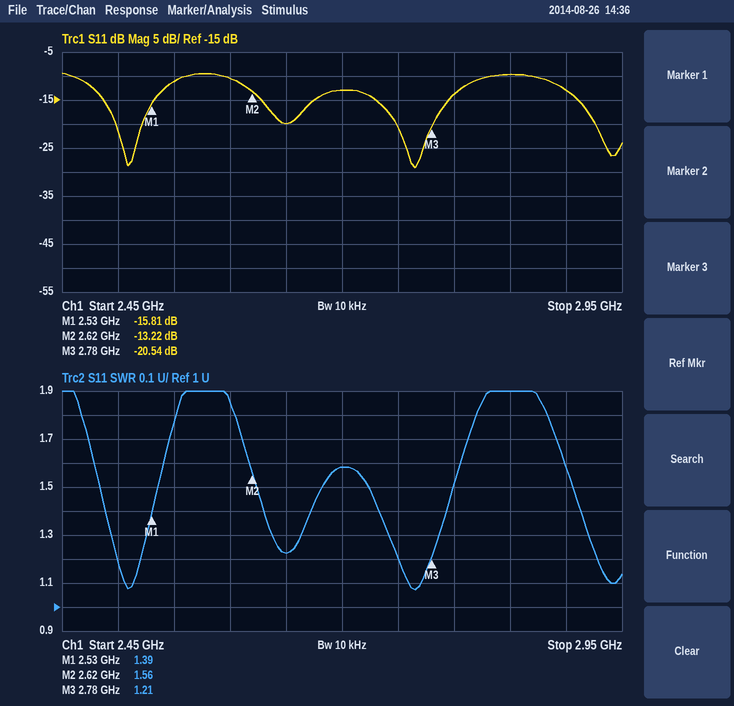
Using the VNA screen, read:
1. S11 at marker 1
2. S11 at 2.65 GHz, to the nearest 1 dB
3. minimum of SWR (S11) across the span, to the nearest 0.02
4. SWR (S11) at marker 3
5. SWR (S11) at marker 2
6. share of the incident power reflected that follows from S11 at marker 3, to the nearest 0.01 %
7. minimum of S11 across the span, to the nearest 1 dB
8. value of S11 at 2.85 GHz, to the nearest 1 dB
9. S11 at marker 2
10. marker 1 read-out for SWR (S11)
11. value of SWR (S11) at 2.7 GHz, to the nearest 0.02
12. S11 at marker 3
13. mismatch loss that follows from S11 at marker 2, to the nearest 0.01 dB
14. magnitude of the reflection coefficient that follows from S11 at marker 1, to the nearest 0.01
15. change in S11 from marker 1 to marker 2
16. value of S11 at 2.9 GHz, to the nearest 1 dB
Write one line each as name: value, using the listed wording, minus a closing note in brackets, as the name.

S11 at marker 1: -15.81 dB
S11 at 2.65 GHz, to the nearest 1 dB: -20 dB
minimum of SWR (S11) across the span, to the nearest 0.02: 1.08
SWR (S11) at marker 3: 1.21
SWR (S11) at marker 2: 1.56
share of the incident power reflected that follows from S11 at marker 3, to the nearest 0.01 %: 0.88 %
minimum of S11 across the span, to the nearest 1 dB: -29 dB
value of S11 at 2.85 GHz, to the nearest 1 dB: -10 dB
S11 at marker 2: -13.22 dB
marker 1 read-out for SWR: 1.39
value of SWR (S11) at 2.7 GHz, to the nearest 0.02: 1.58
S11 at marker 3: -20.54 dB
mismatch loss that follows from S11 at marker 2, to the nearest 0.01 dB: 0.21 dB
magnitude of the reflection coefficient that follows from S11 at marker 1, to the nearest 0.01: 0.16
change in S11 from marker 1 to marker 2: 2.59 dB
value of S11 at 2.9 GHz, to the nearest 1 dB: -13 dB
